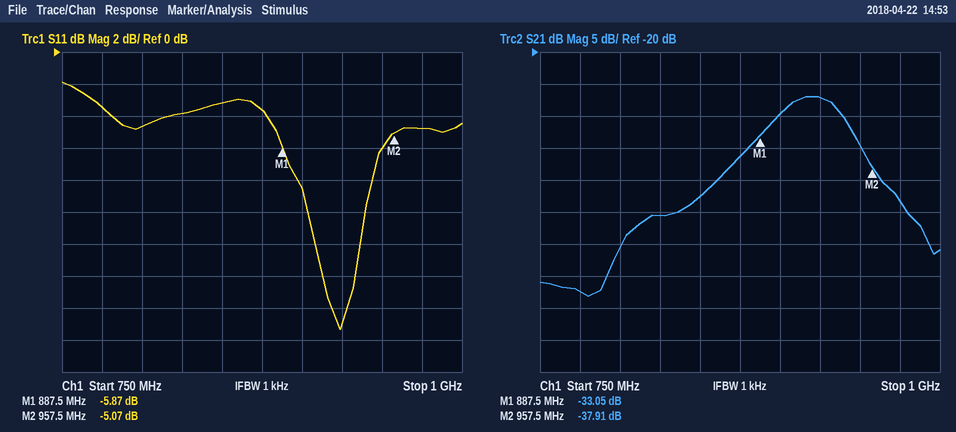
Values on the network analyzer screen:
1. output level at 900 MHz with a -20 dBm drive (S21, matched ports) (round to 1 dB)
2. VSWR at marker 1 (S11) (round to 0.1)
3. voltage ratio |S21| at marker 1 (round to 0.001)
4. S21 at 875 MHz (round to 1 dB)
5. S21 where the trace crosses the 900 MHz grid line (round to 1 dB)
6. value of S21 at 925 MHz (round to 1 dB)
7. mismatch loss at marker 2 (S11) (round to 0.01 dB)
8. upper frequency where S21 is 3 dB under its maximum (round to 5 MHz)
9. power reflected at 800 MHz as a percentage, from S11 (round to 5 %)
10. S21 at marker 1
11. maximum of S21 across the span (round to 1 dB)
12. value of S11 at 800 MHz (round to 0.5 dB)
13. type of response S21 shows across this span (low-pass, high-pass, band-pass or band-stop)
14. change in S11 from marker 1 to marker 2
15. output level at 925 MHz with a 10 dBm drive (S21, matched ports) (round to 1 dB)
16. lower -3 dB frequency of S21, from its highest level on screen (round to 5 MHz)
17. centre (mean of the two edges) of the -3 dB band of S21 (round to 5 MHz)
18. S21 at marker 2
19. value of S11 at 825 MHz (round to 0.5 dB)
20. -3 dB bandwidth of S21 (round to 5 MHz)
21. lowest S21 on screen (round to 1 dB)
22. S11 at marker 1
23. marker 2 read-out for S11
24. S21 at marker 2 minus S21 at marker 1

-50 dBm
3.1
0.022
-36 dB
-30 dB
-27 dB
1.62 dB
940 MHz
35 %
-33.05 dB
-27 dB
-4.5 dB
band-pass
0.80 dB
-17 dBm
900 MHz
920 MHz
-37.91 dB
-4.0 dB
40 MHz
-58 dB
-5.87 dB
-5.07 dB
-4.86 dB
